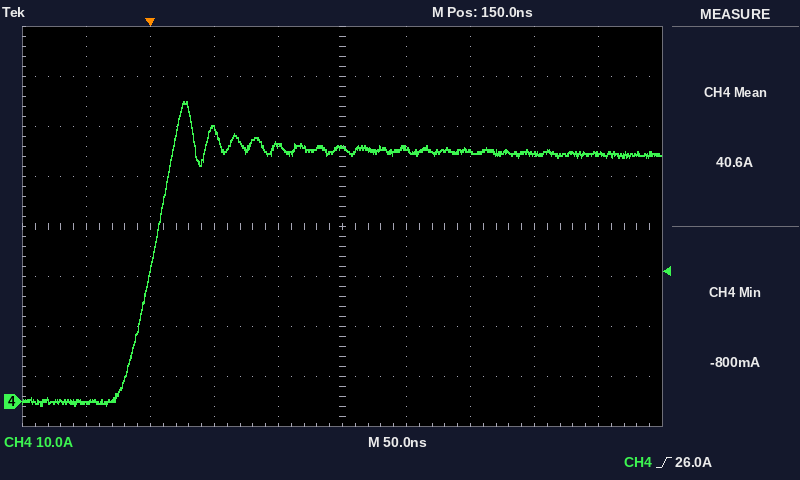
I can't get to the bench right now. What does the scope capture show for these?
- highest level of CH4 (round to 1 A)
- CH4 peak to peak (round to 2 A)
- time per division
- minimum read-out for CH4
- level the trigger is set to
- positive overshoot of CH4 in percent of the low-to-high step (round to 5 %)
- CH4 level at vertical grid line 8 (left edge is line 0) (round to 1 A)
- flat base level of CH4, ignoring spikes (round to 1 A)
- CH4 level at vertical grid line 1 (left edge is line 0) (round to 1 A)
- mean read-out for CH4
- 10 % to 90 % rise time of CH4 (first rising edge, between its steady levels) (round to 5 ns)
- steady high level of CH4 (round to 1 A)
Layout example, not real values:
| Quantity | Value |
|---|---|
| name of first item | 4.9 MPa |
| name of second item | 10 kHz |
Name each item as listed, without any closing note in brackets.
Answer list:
| Quantity | Value |
|---|---|
| highest level of CH4 | 60 A |
| CH4 peak to peak | 60 A |
| time per division | 50 ns |
| minimum read-out for CH4 | -800 mA |
| level the trigger is set to | 26.0 A |
| positive overshoot of CH4 in percent of the low-to-high step | 20 % |
| CH4 level at vertical grid line 8 (left edge is line 0) | 50 A |
| flat base level of CH4, ignoring spikes | 0 A |
| CH4 level at vertical grid line 1 (left edge is line 0) | 0 A |
| mean read-out for CH4 | 40.6 A |
| 10 % to 90 % rise time of CH4 (first rising edge, between its steady levels) | 35 ns |
| steady high level of CH4 | 50 A |
